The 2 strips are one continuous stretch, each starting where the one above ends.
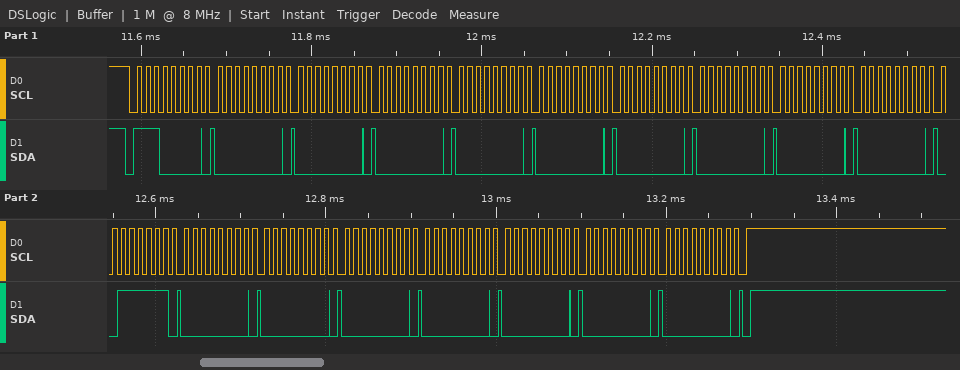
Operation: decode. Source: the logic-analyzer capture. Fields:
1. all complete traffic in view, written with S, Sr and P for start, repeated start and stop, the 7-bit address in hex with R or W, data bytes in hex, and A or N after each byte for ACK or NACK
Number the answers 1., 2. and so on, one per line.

1. S 70W A 00 A 00 A 00 A 00 A 00 A 00 A 00 A 00 A 00 A 3F A 00 A 00 A 00 A 00 A 00 A 00 A 00 A P
